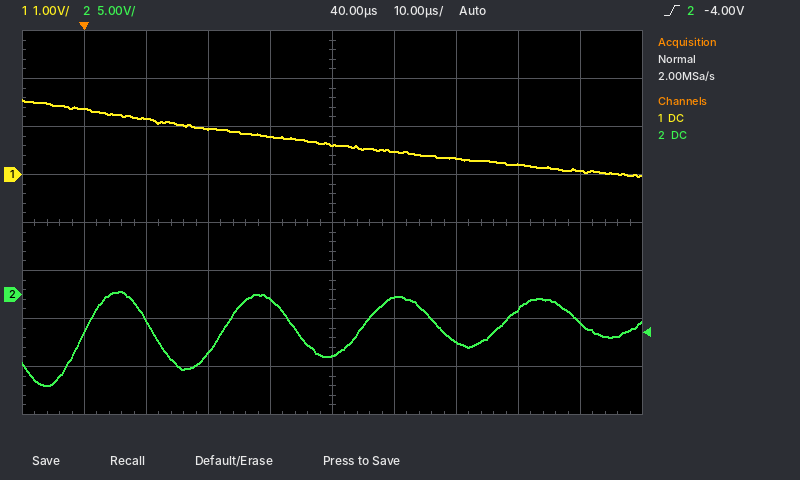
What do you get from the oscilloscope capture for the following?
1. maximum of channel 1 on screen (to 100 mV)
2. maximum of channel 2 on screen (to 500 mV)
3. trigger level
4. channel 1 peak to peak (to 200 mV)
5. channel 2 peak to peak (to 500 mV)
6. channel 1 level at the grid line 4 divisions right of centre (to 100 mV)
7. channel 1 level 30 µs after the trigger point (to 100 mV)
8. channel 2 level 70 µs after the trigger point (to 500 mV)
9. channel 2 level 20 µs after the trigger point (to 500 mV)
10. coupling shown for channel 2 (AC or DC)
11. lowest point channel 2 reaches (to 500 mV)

1.6 V
500 mV
-4.00 V
1.6 V
10.0 V
100 mV
800 mV
-1.5 V
-6.0 V
DC
-9.5 V
